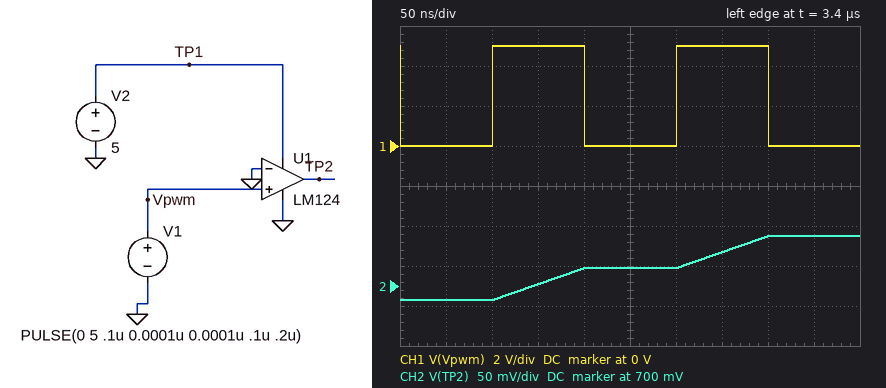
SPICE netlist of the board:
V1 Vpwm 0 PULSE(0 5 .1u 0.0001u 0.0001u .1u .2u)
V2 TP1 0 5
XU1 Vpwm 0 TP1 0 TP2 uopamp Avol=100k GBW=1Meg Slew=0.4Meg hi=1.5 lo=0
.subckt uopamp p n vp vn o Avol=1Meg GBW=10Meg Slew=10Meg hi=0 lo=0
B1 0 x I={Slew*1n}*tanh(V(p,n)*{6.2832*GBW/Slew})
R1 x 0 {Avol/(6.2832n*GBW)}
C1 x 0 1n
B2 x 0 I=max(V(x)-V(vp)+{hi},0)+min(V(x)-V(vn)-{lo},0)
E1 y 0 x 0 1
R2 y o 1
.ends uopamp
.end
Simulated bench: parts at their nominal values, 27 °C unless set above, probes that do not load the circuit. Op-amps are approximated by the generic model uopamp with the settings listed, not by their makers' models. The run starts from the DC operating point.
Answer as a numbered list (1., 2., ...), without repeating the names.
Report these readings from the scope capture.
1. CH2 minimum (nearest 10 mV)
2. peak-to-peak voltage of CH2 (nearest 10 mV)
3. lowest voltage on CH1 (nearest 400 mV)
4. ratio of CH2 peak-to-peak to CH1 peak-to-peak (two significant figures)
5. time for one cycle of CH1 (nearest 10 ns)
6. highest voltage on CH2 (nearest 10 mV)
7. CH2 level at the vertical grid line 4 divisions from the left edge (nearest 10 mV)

1. 680 mV
2. 80 mV
3. 0 V
4. 0.016
5. 200 ns
6. 760 mV
7. 720 mV
